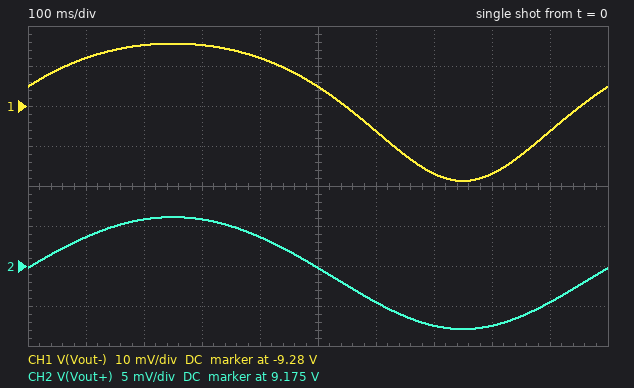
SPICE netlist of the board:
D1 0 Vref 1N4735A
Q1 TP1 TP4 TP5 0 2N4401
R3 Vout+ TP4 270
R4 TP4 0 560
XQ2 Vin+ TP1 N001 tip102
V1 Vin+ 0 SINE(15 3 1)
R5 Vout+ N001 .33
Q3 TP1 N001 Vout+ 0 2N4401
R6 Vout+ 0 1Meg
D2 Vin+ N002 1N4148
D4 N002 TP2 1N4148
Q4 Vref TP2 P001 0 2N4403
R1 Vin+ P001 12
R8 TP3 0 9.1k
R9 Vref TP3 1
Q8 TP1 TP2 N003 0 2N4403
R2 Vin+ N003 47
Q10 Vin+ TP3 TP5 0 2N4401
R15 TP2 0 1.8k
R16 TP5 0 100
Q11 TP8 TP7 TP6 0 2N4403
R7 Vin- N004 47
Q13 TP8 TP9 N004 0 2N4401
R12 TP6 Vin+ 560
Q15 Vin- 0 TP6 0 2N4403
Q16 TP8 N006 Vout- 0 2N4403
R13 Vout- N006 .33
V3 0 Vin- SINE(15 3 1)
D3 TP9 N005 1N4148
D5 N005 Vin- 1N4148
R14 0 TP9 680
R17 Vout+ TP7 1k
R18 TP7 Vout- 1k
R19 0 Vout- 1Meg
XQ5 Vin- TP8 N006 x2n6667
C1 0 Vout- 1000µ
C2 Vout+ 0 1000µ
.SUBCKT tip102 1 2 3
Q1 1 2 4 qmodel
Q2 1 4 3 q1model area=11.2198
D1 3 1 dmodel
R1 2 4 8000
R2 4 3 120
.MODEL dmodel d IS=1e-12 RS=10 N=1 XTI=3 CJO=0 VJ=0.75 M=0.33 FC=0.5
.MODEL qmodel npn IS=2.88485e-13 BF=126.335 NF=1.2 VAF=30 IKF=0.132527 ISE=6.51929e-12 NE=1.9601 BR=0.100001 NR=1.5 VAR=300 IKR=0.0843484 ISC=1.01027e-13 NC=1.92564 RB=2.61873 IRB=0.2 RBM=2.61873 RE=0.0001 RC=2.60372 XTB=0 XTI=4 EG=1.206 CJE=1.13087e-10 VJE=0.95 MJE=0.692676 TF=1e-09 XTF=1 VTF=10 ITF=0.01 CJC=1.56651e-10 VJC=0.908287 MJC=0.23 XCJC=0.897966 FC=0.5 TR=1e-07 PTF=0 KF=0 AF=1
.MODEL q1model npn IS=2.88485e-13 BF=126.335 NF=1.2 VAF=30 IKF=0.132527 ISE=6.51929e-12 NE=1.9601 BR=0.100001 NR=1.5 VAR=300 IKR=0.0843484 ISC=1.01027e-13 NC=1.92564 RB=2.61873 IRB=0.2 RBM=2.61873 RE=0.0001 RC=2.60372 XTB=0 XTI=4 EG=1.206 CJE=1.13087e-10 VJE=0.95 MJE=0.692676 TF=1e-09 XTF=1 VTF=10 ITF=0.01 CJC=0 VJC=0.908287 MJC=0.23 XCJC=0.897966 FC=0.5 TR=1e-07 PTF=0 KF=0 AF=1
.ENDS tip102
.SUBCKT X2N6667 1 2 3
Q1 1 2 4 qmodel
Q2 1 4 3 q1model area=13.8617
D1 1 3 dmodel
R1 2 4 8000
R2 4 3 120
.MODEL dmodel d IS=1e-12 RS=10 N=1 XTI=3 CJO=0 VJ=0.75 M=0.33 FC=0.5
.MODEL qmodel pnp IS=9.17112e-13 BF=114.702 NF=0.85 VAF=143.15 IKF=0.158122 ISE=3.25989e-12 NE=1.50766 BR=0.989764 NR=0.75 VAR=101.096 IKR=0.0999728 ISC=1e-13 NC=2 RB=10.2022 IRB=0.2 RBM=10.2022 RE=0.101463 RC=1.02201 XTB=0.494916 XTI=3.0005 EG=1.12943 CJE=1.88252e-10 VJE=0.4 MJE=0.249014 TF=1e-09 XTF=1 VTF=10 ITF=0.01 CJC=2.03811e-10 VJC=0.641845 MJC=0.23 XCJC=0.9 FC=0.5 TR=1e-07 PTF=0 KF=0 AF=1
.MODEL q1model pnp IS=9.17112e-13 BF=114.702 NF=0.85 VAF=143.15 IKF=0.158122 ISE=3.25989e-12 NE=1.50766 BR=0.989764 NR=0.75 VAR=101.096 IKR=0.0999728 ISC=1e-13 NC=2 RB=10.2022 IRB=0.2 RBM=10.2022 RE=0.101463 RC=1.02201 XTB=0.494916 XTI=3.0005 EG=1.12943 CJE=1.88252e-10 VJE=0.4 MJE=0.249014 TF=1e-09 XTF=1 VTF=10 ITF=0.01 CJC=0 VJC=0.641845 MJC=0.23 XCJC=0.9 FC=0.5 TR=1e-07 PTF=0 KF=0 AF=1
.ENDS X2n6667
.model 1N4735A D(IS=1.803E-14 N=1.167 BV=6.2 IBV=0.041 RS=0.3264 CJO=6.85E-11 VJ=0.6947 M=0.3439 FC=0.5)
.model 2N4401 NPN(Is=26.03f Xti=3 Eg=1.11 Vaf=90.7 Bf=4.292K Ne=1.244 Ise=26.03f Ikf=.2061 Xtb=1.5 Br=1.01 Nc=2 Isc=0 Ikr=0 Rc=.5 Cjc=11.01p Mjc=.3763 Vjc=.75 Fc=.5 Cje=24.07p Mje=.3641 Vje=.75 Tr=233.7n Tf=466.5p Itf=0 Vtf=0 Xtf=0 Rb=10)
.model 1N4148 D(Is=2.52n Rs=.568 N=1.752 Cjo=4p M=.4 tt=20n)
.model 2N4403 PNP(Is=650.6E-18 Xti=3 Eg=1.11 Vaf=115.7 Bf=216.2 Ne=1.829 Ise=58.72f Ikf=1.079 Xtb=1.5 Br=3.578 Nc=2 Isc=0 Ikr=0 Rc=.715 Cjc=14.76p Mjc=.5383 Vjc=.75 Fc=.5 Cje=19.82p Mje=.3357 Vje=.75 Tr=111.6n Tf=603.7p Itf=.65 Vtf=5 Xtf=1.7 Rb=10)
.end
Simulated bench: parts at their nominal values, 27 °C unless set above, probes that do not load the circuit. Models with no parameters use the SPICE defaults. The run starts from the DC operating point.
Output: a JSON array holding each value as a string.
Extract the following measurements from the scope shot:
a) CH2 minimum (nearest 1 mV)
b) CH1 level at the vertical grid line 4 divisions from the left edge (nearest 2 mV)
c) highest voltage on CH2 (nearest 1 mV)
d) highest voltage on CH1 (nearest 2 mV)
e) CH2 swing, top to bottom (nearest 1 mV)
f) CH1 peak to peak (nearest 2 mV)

["9.167 V", "-9.268 V", "9.181 V", "-9.264 V", "14 mV", "34 mV"]
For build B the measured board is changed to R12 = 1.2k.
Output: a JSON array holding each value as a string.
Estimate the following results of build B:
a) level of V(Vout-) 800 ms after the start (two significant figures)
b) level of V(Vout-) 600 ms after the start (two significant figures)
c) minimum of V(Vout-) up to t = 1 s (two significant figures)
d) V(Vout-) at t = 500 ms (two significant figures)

["-11 V", "-13 V", "-15 V", "-14 V"]
